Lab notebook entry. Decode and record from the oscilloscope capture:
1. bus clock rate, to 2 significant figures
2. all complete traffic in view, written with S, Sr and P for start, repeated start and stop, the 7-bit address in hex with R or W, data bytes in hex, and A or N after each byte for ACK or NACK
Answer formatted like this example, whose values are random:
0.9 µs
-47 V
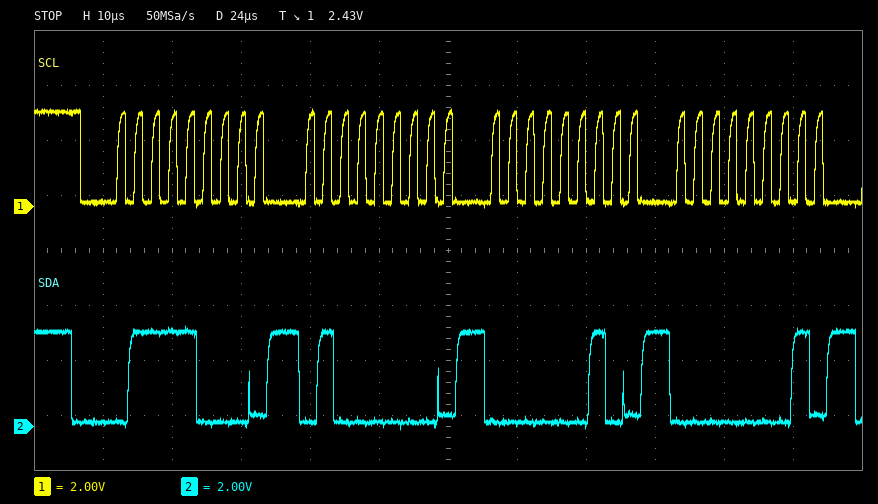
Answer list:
400 kHz
S 3CW A 40 A 02 A 01 A
